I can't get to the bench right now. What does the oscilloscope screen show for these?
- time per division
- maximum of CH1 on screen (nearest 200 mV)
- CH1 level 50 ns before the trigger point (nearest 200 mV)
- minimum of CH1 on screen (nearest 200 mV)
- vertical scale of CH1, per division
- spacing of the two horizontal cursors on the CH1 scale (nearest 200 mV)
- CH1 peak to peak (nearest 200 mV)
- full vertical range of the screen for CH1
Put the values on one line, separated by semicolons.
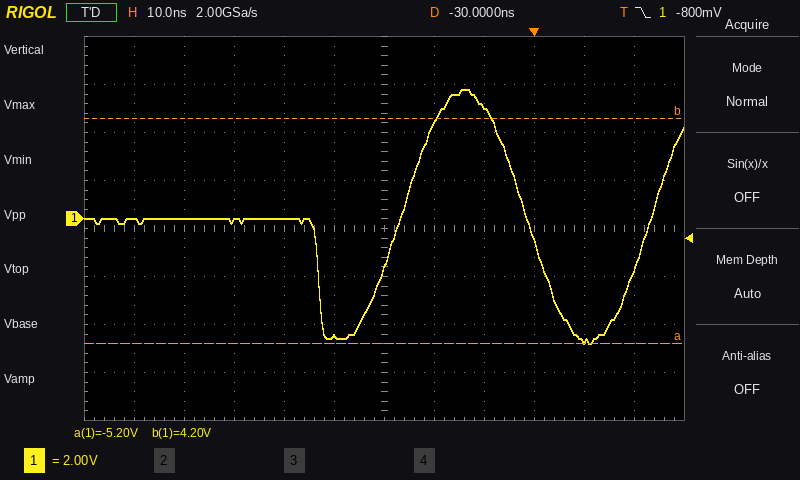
10 ns; 5.4 V; 0.0 V; -5.2 V; 2 V; 9.4 V; 10.6 V; 16 V
